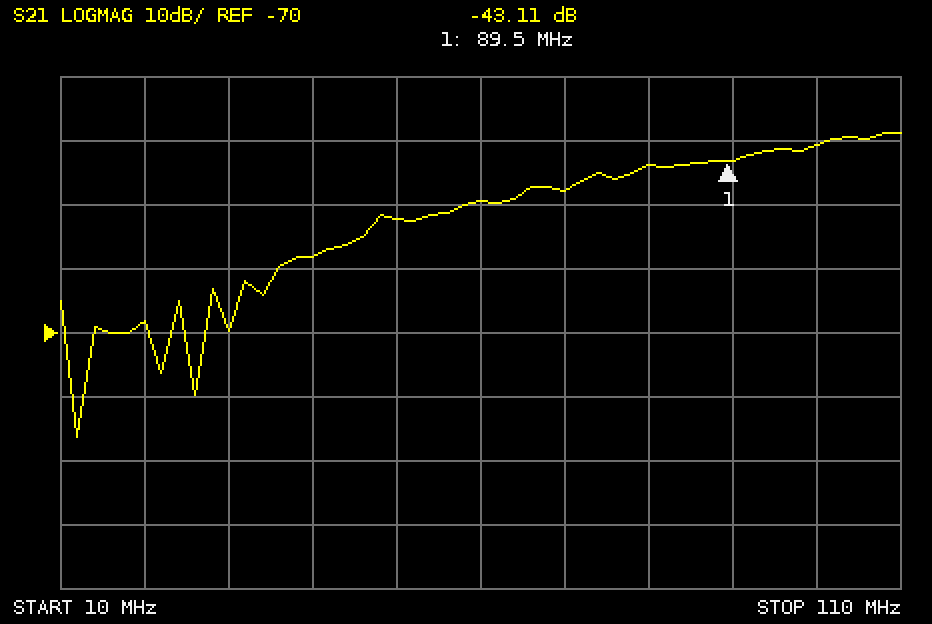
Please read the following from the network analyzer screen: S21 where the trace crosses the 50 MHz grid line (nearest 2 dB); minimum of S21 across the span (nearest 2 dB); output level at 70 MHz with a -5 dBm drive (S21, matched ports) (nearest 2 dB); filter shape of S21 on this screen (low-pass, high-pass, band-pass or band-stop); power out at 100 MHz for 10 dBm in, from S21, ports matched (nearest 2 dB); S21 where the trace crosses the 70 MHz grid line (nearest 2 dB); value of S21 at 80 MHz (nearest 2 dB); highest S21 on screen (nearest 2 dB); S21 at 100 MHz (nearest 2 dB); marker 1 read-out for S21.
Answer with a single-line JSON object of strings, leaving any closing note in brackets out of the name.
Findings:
{"S21 where the trace crosses the 50 MHz grid line": "-52 dB", "minimum of S21 across the span": "-86 dB", "output level at 70 MHz with a -5 dBm drive (S21, matched ports)": "-52 dBm", "filter shape of S21 on this screen": "high-pass", "power out at 100 MHz for 10 dBm in, from S21, ports matched": "-30 dBm", "S21 where the trace crosses the 70 MHz grid line": "-48 dB", "value of S21 at 80 MHz": "-44 dB", "highest S21 on screen": "-38 dB", "S21 at 100 MHz": "-40 dB", "marker 1 read-out for S21": "-43.11 dB"}
